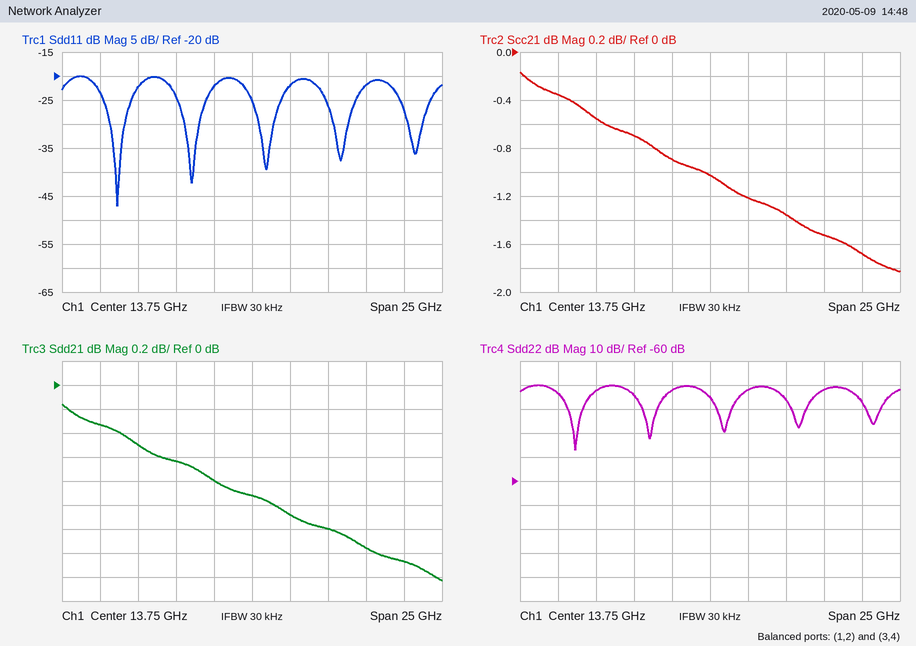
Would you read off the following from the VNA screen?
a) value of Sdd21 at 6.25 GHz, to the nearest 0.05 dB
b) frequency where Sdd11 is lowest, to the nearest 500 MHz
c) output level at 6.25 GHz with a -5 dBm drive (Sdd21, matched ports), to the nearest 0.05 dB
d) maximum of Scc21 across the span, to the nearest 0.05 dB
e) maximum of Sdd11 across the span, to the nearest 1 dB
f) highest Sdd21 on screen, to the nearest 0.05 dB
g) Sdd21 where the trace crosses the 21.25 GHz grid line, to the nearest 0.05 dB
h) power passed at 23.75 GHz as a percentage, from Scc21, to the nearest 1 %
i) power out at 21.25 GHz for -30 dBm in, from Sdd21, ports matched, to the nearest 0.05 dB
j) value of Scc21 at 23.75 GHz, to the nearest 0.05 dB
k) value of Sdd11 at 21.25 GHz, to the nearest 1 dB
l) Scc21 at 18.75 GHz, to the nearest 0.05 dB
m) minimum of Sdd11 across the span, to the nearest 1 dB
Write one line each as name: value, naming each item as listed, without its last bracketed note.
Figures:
value of Sdd21 at 6.25 GHz, to the nearest 0.05 dB: -0.50 dB
frequency where Sdd11 is lowest, to the nearest 500 MHz: 5.0 GHz
output level at 6.25 GHz with a -5 dBm drive (Sdd21, matched ports), to the nearest 0.05 dB: -5.50 dBm
maximum of Scc21 across the span, to the nearest 0.05 dB: -0.15 dB
maximum of Sdd11 across the span, to the nearest 1 dB: -20 dB
highest Sdd21 on screen, to the nearest 0.05 dB: -0.15 dB
Sdd21 where the trace crosses the 21.25 GHz grid line, to the nearest 0.05 dB: -1.35 dB
power passed at 23.75 GHz as a percentage, from Scc21, to the nearest 1 %: 68 %
power out at 21.25 GHz for -30 dBm in, from Sdd21, ports matched, to the nearest 0.05 dB: -31.35 dBm
value of Scc21 at 23.75 GHz, to the nearest 0.05 dB: -1.70 dB
value of Sdd11 at 21.25 GHz, to the nearest 1 dB: -22 dB
Scc21 at 18.75 GHz, to the nearest 0.05 dB: -1.35 dB
minimum of Sdd11 across the span, to the nearest 1 dB: -47 dB
